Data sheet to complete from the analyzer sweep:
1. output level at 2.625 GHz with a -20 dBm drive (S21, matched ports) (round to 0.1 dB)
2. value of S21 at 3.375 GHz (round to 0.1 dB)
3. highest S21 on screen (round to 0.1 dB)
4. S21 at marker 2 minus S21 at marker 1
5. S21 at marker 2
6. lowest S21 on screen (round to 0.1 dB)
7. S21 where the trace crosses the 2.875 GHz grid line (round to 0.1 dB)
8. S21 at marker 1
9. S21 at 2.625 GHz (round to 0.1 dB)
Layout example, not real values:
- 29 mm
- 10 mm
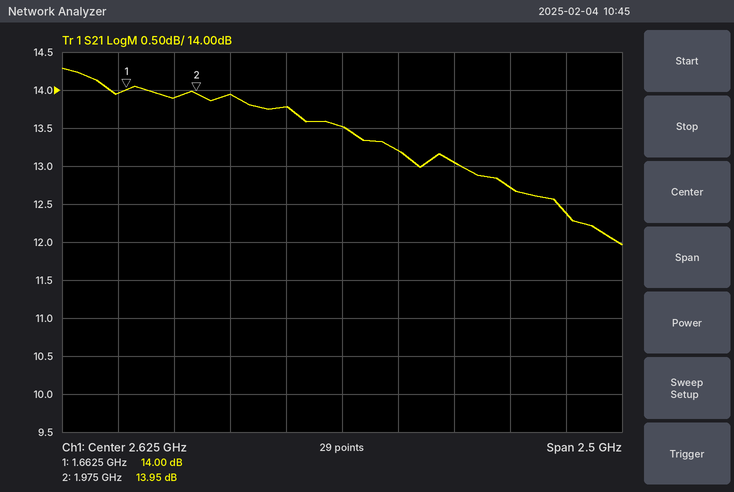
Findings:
- -6.5 dBm
- 12.7 dB
- 14.3 dB
- -0.05 dB
- 13.95 dB
- 12.0 dB
- 13.2 dB
- 14.00 dB
- 13.5 dB
